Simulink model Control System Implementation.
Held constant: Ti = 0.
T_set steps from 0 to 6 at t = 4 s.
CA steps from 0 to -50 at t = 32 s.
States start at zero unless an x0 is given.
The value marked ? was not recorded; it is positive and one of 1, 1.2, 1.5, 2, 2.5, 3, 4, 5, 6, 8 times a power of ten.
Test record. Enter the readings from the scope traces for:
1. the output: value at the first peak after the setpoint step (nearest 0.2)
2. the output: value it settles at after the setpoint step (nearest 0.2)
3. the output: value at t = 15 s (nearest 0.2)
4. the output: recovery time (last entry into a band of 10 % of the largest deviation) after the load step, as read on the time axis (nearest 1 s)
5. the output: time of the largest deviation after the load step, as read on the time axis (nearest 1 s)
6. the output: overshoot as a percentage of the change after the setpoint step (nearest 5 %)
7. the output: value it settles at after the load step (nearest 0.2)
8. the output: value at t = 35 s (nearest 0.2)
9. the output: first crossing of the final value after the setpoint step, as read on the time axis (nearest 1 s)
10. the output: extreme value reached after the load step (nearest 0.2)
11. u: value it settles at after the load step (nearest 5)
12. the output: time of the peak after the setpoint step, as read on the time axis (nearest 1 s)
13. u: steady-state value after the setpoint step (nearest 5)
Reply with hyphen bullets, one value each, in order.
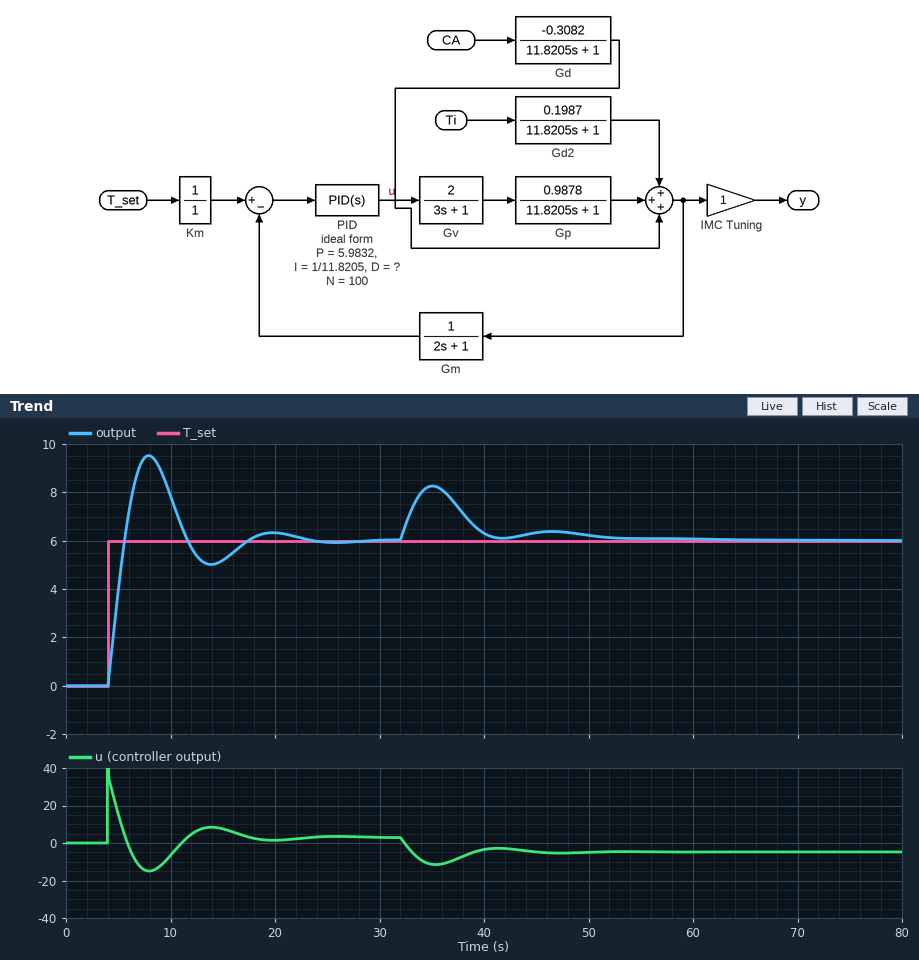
- 9.6
- 6.0
- 5.2
- 50 s
- 35 s
- 60 %
- 6.0
- 8.2
- 6 s
- 8.2
- -5
- 8 s
- 5
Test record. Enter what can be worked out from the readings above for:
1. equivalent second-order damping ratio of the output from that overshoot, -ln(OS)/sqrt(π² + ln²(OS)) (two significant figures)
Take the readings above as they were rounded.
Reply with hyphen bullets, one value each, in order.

- 0.16
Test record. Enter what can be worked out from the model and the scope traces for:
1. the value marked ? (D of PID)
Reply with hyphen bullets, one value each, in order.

- 2
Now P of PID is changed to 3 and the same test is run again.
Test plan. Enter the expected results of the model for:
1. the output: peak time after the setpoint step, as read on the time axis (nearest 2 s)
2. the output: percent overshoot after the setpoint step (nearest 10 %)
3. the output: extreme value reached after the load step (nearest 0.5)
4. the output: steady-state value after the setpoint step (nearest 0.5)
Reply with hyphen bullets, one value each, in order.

- 10 s
- 30 %
- 9.0
- 6.0
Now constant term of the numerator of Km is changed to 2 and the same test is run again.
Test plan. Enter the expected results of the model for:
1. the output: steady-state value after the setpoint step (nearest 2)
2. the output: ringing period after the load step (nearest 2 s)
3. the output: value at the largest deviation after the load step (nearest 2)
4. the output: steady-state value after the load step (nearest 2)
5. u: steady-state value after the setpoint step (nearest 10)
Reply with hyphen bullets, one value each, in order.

- 12
- 12 s
- 14
- 12
- 10
